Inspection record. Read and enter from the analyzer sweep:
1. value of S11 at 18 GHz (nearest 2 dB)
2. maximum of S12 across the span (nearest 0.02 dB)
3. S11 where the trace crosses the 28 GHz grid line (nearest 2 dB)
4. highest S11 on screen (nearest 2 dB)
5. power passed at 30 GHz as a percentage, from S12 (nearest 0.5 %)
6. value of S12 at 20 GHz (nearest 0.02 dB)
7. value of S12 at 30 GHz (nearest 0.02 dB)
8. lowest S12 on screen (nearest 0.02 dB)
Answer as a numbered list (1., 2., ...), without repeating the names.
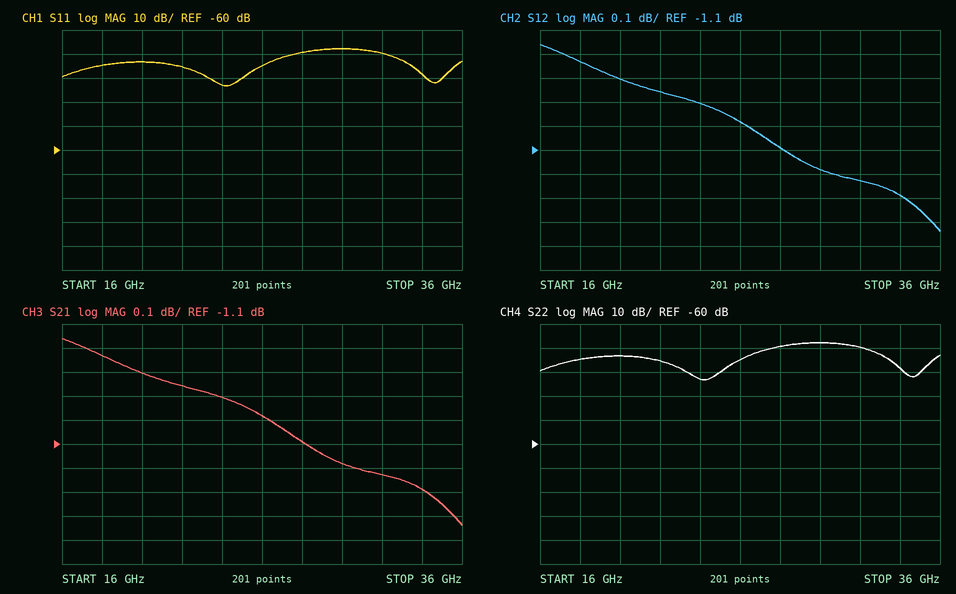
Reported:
1. -24 dB
2. -0.66 dB
3. -20 dB
4. -18 dB
5. 76.0 %
6. -0.80 dB
7. -1.18 dB
8. -1.44 dB
